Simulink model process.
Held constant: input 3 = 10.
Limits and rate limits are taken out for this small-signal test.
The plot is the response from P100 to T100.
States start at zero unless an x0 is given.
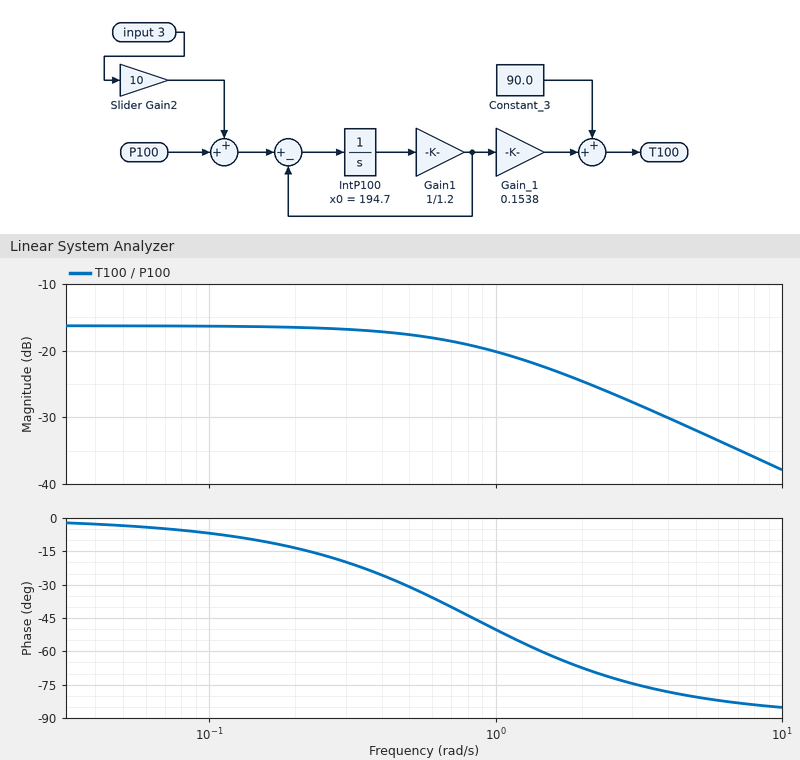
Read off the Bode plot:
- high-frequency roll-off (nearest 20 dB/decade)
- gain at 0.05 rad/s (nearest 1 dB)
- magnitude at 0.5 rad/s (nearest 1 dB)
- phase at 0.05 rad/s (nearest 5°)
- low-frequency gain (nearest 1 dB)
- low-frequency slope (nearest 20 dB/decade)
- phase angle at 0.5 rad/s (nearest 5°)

-20 dB/decade
-16 dB
-18 dB
-5°
-16 dB
0 dB/decade
-30°
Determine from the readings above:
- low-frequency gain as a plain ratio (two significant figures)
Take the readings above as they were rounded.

0.16
